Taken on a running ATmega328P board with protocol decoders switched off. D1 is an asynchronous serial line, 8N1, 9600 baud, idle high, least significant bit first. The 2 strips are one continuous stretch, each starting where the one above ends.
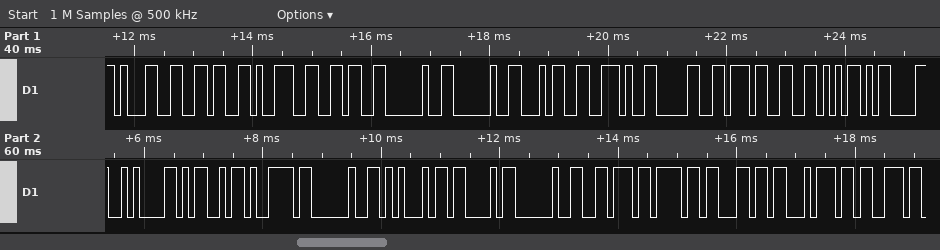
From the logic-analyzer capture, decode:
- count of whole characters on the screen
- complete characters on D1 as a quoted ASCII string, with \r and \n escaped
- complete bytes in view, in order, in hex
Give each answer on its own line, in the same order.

24
"1696  4.07V\r\nMy EC volts"
31 36 39 36 20 20 34 2E 30 37 56 0D 0A 4D 79 20 45 43 20 76 6F 6C 74 73
